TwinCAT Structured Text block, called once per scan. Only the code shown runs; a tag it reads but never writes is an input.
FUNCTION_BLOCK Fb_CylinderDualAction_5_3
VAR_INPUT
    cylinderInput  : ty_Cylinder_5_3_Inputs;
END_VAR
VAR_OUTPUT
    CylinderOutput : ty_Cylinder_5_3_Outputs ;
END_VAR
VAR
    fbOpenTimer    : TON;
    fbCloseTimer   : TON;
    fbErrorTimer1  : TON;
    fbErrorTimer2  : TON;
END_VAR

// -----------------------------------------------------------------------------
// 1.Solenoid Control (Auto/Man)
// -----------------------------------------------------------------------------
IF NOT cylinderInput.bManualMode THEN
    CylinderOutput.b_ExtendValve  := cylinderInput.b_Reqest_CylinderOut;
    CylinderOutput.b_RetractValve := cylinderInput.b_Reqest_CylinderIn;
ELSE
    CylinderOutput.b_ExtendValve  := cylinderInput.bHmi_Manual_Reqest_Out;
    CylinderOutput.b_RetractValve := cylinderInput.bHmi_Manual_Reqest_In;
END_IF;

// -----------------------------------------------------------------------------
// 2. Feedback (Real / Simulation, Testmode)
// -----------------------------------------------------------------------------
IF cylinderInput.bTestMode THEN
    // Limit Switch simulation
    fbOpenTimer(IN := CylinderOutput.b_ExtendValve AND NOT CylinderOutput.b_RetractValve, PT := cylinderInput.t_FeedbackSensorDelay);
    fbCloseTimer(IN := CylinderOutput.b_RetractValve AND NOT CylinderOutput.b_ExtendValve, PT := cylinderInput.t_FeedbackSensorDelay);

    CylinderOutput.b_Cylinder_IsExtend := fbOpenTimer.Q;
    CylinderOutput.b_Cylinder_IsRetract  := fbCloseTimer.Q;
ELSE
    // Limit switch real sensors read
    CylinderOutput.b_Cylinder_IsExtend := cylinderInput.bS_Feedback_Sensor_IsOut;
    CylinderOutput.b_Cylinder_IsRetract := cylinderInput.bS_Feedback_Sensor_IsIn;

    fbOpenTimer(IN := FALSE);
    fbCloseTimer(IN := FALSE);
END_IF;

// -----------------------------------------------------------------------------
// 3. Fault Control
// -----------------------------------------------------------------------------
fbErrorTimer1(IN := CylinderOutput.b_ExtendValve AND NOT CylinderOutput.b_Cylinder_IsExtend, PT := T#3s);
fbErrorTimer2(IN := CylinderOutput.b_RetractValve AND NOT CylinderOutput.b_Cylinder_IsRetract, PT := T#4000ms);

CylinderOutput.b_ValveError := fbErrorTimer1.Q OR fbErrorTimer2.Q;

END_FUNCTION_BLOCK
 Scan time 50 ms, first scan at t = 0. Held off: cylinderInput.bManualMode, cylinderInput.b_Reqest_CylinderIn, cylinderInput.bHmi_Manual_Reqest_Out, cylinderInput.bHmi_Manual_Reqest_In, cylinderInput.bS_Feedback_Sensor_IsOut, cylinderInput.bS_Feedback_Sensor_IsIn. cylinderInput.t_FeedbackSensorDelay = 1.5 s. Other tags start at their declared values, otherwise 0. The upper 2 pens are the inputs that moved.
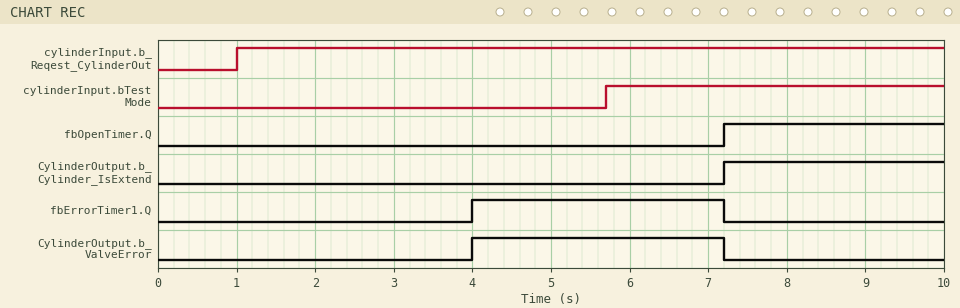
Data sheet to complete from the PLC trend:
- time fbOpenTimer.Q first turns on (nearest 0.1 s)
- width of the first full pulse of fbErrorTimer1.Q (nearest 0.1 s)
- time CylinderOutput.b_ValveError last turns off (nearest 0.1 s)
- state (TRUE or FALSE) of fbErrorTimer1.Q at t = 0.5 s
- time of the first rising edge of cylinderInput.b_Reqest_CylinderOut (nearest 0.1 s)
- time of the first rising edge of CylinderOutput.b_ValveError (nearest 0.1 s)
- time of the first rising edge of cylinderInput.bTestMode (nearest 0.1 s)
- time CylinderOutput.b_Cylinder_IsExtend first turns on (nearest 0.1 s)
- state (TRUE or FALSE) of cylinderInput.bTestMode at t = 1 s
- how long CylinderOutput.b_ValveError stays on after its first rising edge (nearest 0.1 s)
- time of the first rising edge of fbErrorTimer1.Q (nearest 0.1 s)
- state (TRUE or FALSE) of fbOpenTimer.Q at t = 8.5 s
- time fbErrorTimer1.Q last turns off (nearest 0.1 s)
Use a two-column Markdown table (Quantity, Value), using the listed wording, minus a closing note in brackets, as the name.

| Quantity | Value |
|---|---|
| time fbOpenTimer.Q first turns on | 7.2 s |
| width of the first full pulse of fbErrorTimer1.Q | 3.2 s |
| time CylinderOutput.b_ValveError last turns off | 7.2 s |
| state (TRUE or FALSE) of fbErrorTimer1.Q at t = 0.5 s | FALSE |
| time of the first rising edge of cylinderInput.b_Reqest_CylinderOut | 1.0 s |
| time of the first rising edge of CylinderOutput.b_ValveError | 4.0 s |
| time of the first rising edge of cylinderInput.bTestMode | 5.7 s |
| time CylinderOutput.b_Cylinder_IsExtend first turns on | 7.2 s |
| state (TRUE or FALSE) of cylinderInput.bTestMode at t = 1 s | FALSE |
| how long CylinderOutput.b_ValveError stays on after its first rising edge | 3.2 s |
| time of the first rising edge of fbErrorTimer1.Q | 4.0 s |
| state (TRUE or FALSE) of fbOpenTimer.Q at t = 8.5 s | TRUE |
| time fbErrorTimer1.Q last turns off | 7.2 s |
